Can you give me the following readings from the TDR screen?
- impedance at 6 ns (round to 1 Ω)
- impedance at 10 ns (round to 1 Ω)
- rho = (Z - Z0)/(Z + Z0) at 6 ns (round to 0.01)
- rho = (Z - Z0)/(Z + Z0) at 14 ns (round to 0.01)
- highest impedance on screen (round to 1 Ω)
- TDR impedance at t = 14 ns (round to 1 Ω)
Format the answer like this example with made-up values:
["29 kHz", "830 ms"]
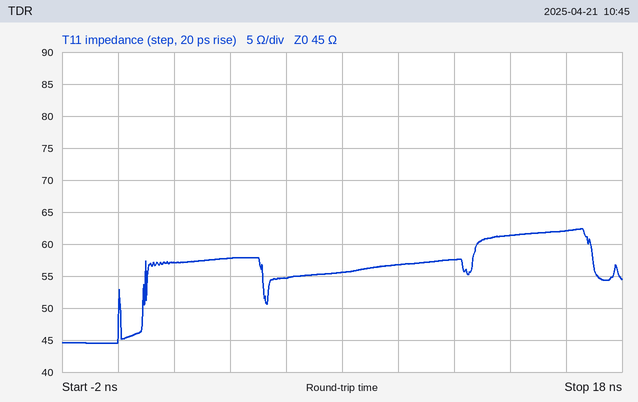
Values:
["55 Ω", "57 Ω", "+0.10", "+0.15", "62 Ω", "61 Ω"]
